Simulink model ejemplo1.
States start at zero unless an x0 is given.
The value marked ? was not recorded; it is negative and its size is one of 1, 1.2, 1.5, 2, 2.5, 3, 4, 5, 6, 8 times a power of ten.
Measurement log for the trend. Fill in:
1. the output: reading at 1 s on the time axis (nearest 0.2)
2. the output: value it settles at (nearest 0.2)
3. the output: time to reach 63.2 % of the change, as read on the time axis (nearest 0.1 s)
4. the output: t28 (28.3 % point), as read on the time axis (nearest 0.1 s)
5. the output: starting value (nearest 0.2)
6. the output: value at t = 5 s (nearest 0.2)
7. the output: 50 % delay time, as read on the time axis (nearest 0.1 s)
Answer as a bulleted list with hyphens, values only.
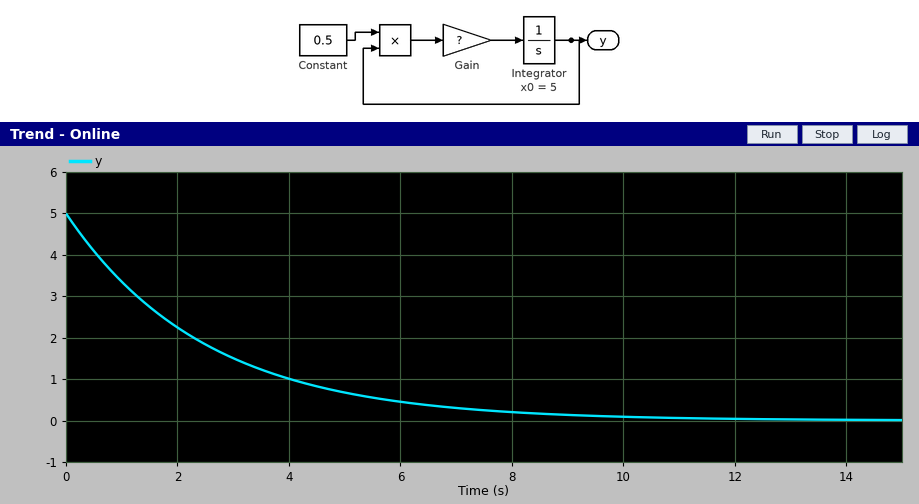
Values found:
- 3.4
- 0.0
- 2.5 s
- 0.8 s
- 5.0
- 0.6
- 1.7 s
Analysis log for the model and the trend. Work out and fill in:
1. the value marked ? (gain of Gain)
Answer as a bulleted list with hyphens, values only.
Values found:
- -0.8
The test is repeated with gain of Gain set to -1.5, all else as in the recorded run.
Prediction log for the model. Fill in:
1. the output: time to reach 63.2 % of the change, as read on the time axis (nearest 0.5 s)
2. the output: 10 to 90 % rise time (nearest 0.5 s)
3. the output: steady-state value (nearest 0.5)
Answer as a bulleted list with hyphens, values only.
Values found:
- 1.5 s
- 3.0 s
- 0.0
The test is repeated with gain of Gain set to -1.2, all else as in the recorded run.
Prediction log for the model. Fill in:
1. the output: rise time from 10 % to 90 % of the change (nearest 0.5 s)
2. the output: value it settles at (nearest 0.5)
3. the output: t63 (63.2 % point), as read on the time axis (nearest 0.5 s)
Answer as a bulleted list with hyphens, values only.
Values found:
- 3.5 s
- 0.0
- 1.5 s
